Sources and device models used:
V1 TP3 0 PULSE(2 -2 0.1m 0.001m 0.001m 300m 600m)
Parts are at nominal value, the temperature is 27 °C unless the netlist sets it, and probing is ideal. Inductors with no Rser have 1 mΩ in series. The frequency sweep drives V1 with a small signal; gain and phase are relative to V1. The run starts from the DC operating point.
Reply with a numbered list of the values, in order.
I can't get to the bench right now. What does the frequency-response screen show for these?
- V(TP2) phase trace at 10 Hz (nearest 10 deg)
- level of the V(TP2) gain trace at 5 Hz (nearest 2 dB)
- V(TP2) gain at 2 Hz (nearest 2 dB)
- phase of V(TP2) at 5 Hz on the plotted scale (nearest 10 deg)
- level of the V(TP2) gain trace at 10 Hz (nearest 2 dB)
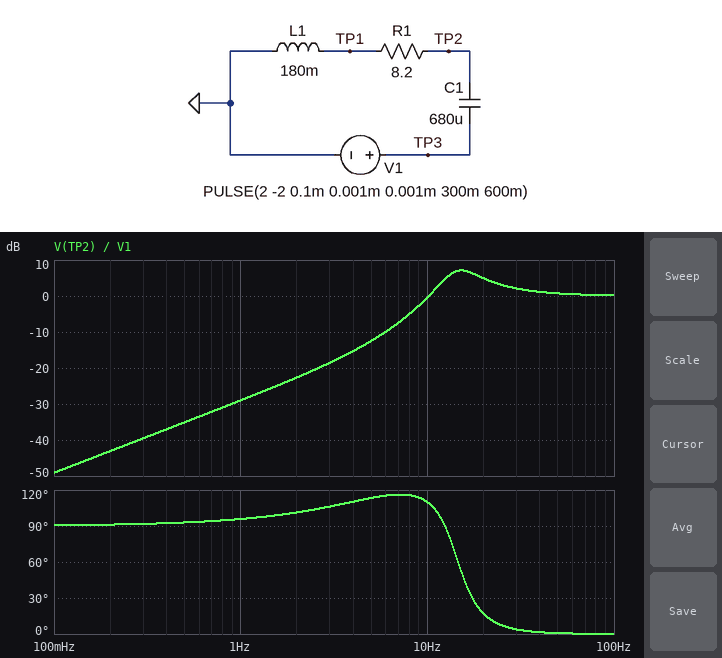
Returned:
1. 110 deg
2. -12 dB
3. -22 dB
4. 110 deg
5. 0 dB
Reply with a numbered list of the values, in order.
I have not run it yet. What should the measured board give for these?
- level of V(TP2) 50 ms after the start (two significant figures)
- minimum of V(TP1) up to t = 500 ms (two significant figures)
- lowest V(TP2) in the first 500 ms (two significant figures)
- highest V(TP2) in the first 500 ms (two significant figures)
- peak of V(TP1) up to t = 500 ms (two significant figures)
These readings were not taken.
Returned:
1. 750 mV
2. -4.0 V
3. -4.0 V
4. 4.0 V
5. 4.0 V
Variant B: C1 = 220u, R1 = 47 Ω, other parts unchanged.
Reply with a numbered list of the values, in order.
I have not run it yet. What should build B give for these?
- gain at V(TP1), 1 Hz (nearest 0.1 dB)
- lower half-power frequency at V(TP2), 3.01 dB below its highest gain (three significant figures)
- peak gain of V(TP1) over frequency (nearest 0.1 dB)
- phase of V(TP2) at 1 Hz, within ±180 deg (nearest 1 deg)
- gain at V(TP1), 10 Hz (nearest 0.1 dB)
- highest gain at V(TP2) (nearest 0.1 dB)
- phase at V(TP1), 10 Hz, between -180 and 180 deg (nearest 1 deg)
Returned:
1. -56.1 dB
2. 14.4 Hz
3. 0 dB
4. 88 deg
5. -16.7 dB
6. 1.7 dB
7. 142 deg
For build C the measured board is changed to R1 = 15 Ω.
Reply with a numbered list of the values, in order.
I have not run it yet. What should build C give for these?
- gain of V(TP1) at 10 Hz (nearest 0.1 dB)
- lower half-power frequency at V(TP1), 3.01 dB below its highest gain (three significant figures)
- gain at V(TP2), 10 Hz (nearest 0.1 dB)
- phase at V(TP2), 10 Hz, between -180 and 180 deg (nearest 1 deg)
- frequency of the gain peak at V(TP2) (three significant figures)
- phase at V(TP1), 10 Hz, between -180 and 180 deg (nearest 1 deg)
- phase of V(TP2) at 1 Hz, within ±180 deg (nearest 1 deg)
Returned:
1. -4.6 dB
2. 12.2 Hz
3. -0.2 dB
4. 76 deg
5. 16.5 Hz
6. 129 deg
7. 91 deg
